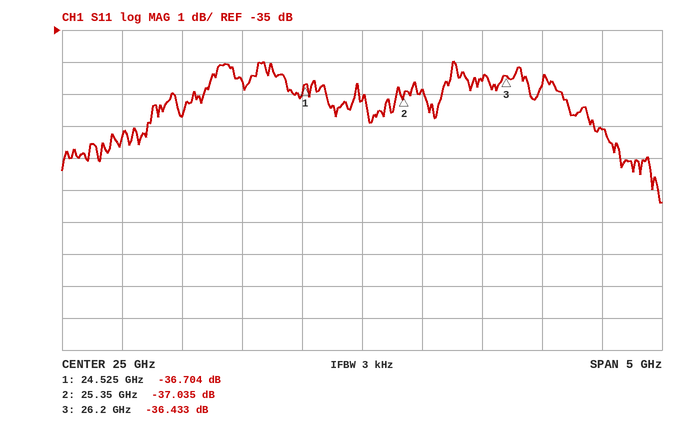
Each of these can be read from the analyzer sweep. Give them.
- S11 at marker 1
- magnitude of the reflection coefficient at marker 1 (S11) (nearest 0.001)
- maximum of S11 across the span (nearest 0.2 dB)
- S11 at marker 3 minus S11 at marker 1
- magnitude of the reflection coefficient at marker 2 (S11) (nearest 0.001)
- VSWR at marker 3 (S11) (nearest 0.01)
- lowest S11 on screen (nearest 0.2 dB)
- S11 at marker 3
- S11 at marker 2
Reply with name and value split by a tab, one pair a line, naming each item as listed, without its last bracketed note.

S11 at marker 1	-36.704 dB
magnitude of the reflection coefficient at marker 1 (S11)	0.015
maximum of S11 across the span	-36.0 dB
S11 at marker 3 minus S11 at marker 1	0.271 dB
magnitude of the reflection coefficient at marker 2 (S11)	0.014
VSWR at marker 3 (S11)	1.03
lowest S11 on screen	-40.4 dB
S11 at marker 3	-36.433 dB
S11 at marker 2	-37.035 dB
